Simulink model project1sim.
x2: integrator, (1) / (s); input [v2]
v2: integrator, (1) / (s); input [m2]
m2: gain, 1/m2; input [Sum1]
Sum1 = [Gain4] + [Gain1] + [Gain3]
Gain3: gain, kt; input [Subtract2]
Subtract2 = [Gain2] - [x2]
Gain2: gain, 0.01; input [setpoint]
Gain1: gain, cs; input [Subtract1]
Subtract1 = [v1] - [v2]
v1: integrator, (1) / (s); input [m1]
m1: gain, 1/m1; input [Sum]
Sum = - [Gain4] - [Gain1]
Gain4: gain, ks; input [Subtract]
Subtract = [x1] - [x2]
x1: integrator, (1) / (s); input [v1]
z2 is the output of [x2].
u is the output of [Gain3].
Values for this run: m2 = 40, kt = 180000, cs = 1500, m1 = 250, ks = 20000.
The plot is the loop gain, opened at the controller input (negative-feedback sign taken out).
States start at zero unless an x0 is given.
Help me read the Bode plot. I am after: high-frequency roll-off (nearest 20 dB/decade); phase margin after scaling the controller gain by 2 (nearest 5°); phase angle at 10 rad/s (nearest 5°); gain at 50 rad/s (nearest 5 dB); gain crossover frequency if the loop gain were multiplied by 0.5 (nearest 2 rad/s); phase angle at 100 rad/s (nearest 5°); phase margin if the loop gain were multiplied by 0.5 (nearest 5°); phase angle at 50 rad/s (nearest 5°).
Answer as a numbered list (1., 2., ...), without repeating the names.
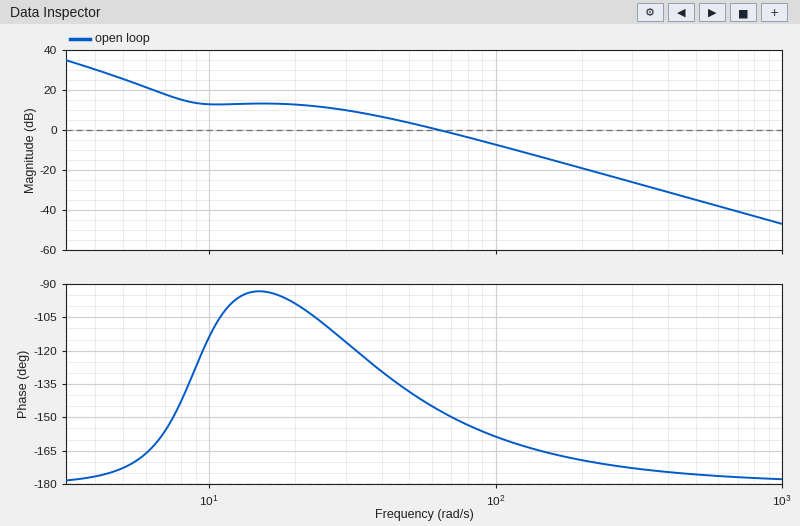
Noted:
1. -40 dB/decade
2. 25°
3. -115°
4. 5 dB
5. 42 rad/s
6. -160°
7. 50°
8. -140°
